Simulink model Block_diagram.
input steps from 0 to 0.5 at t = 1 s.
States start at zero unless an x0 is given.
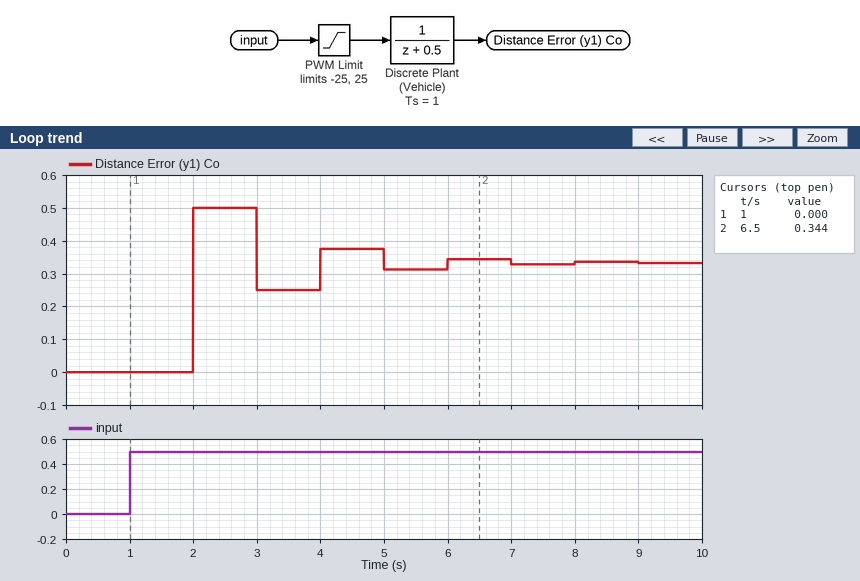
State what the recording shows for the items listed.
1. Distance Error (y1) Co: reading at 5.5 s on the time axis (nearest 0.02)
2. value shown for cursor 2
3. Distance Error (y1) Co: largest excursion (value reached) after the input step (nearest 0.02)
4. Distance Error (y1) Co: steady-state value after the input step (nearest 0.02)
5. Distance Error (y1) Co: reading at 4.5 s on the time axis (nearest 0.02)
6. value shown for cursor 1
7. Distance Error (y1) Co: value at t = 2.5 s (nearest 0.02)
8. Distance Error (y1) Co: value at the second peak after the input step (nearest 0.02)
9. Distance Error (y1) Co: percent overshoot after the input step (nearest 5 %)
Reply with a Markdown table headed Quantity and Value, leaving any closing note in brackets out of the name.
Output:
| Quantity | Value |
|---|---|
| Distance Error (y1) Co: reading at 5.5 s on the time axis | 0.32 |
| value shown for cursor 2 | 0.344 |
| Distance Error (y1) Co: largest excursion (value reached) after the input step | 0.50 |
| Distance Error (y1) Co: steady-state value after the input step | 0.34 |
| Distance Error (y1) Co: reading at 4.5 s on the time axis | 0.38 |
| value shown for cursor 1 | 0.000 |
| Distance Error (y1) Co: value at t = 2.5 s | 0.50 |
| Distance Error (y1) Co: value at the second peak after the input step | 0.38 |
| Distance Error (y1) Co: percent overshoot after the input step | 50 % |
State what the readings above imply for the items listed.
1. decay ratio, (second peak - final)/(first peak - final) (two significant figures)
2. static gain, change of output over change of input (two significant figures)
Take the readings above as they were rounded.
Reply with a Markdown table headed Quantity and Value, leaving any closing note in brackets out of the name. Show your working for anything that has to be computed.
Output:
| Quantity | Value |
|---|---|
| decay ratio, (second peak - final)/(first peak - final) | (0.38 - 0.34) / (0.5 - 0.34) = 0.25 |
| static gain, change of output over change of input | (0.34 - 0) / (0.5 - 0) = 0.68 |
